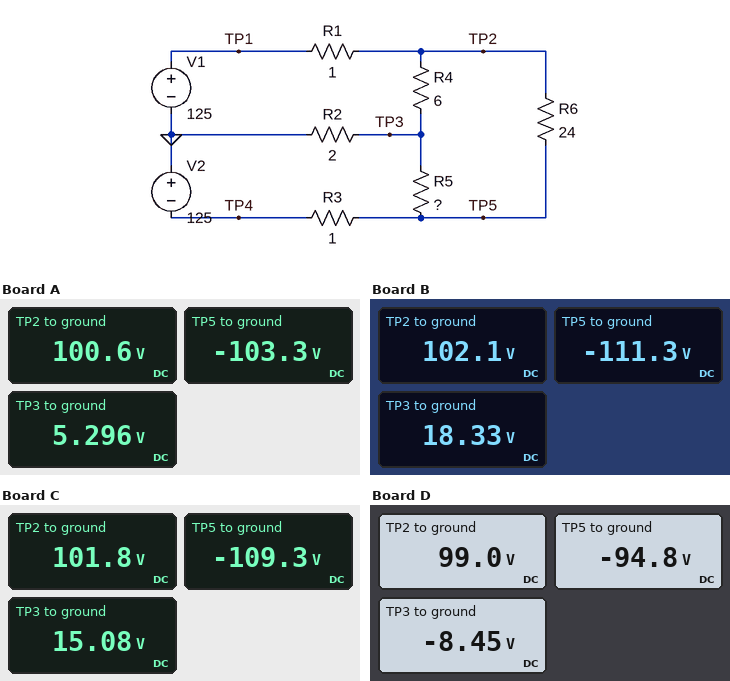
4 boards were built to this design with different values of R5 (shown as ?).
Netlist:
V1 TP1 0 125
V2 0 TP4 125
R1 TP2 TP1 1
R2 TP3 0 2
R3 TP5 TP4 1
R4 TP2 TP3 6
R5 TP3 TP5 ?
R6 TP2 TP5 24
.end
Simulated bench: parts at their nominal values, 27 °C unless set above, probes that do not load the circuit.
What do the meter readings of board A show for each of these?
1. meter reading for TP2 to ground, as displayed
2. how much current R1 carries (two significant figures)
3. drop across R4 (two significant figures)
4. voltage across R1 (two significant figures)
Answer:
100.6 V
24 A
95 V
24 V
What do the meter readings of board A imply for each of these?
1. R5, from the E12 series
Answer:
8.2 Ω
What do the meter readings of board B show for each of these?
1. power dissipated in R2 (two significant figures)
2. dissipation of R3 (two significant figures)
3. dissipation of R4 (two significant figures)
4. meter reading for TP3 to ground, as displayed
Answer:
170 W
190 W
1.2 kW
18.33 V
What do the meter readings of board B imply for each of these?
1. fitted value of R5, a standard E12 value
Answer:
27 Ω
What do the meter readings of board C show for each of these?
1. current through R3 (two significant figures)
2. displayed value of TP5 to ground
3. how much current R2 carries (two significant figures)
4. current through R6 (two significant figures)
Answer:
16 A
-109.3 V
7.5 A
8.8 A
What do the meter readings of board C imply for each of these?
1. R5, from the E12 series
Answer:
18 Ω
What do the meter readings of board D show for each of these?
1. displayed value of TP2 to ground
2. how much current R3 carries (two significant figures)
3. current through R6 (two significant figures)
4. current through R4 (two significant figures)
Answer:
99.0 V
30 A
8.1 A
18 A
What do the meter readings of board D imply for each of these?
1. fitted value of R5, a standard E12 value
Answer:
3.9 Ω
